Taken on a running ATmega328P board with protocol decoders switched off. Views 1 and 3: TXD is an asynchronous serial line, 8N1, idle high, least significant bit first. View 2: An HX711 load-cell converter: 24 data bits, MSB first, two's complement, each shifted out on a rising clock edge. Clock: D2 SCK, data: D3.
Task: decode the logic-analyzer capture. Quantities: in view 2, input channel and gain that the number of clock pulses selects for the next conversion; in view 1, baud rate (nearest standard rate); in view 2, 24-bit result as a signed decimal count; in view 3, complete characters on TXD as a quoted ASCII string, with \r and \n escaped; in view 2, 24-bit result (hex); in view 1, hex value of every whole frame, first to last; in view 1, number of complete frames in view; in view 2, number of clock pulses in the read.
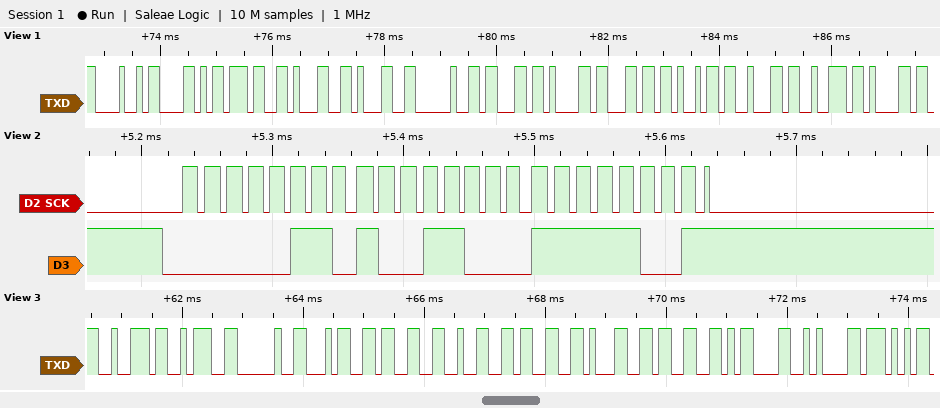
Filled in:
channel A, gain 128
9600 baud
432377
"r: 432313\r\nW"
0x0698F9
48 58 37 31 31 20 63 61 6C 69 62 72 61
13
25
